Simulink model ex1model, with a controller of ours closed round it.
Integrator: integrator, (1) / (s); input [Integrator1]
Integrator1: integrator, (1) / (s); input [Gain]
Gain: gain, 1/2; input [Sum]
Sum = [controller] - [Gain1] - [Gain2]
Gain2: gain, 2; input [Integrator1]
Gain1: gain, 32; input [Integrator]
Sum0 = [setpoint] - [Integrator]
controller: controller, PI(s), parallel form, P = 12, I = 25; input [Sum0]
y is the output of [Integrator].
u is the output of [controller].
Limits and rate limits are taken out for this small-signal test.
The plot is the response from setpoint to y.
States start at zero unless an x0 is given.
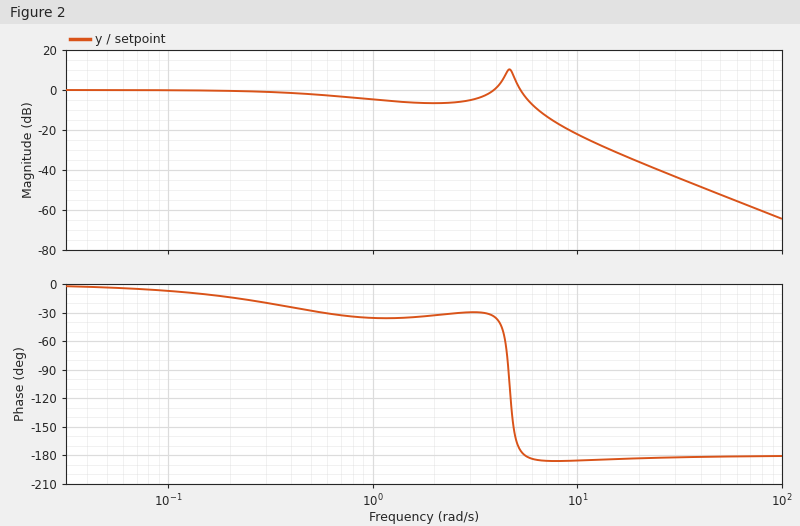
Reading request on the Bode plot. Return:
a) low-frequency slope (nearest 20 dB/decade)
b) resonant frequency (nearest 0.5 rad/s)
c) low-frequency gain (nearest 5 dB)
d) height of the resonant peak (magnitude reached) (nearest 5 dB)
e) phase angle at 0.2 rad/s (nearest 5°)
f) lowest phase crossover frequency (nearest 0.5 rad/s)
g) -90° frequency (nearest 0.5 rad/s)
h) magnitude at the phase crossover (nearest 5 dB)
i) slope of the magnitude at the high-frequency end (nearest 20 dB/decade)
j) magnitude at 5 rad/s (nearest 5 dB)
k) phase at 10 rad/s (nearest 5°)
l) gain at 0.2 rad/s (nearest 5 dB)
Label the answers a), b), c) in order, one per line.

a) 0 dB/decade
b) 4.5 rad/s
c) 0 dB
d) 10 dB
e) -15°
f) 5.5 rad/s
g) 4.5 rad/s
h) -5 dB
i) -40 dB/decade
j) 5 dB
k) -185°
l) 0 dB
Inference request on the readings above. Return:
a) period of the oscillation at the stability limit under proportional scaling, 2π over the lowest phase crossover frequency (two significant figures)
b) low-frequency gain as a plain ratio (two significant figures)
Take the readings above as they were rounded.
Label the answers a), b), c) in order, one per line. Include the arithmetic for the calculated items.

a) 2π / 5.5 = 1.1 s
b) 10^(0 / 20) = 1.0
